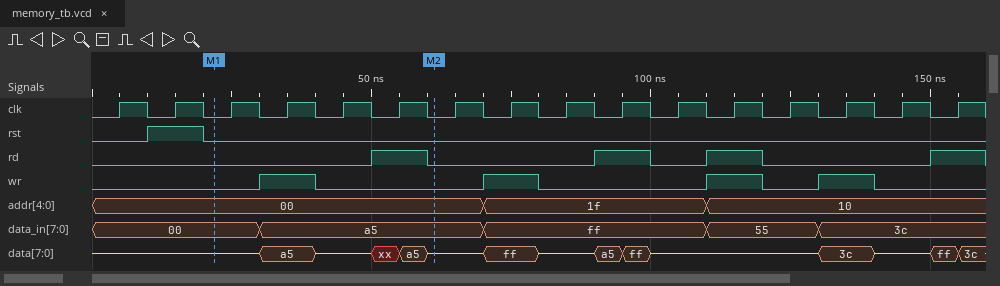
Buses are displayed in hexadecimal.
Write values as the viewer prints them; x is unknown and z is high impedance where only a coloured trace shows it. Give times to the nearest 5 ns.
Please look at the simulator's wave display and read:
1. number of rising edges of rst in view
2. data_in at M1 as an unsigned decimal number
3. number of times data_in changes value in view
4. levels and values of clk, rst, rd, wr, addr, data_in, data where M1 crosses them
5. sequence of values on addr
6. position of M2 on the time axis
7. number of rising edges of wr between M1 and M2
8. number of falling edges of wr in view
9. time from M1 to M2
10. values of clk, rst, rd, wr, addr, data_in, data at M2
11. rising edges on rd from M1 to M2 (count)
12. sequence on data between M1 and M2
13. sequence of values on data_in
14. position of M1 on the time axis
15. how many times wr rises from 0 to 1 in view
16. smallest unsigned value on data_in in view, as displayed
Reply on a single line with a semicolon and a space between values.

1; 0; 4; clk=0, rst=0, rd=0, wr=0, addr=00, data_in=00, data=z; 00, 1f, 10; 60 ns; 1; 4; 40 ns; clk=0, rst=0, rd=0, wr=0, addr=00, data_in=a5, data=z; 1; z, a5, z, xx, a5, z; 00, a5, ff, 55, 3c; 20 ns; 4; 00
